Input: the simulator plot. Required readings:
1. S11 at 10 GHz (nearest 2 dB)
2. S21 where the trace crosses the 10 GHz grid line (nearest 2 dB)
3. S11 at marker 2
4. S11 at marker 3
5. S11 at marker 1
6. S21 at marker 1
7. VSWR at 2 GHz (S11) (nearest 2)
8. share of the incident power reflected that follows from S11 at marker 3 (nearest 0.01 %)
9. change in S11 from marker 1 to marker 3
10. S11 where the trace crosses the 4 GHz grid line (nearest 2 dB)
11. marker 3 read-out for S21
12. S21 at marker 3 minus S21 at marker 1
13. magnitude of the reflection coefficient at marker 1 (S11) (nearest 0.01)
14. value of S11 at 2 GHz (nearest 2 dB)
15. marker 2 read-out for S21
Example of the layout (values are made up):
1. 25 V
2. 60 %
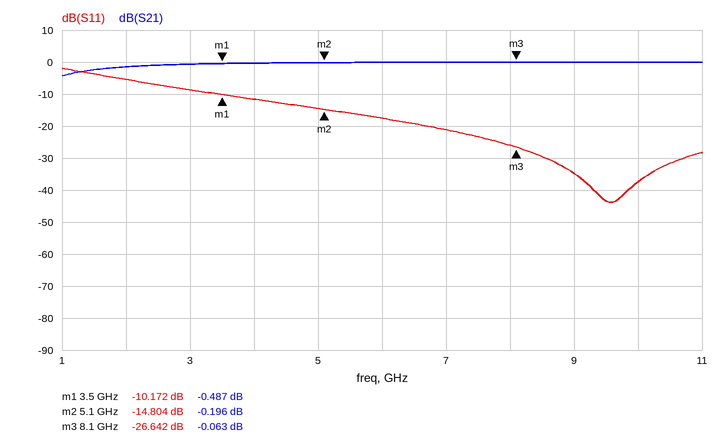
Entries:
1. -38 dB
2. 0 dB
3. -14.804 dB
4. -26.642 dB
5. -10.172 dB
6. -0.487 dB
7. 4
8. 0.22 %
9. -16.470 dB
10. -12 dB
11. -0.063 dB
12. 0.424 dB
13. 0.31
14. -6 dB
15. -0.196 dB
